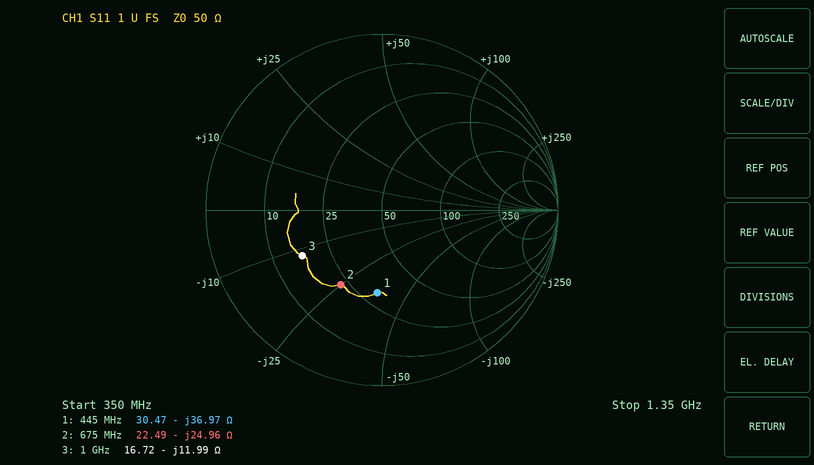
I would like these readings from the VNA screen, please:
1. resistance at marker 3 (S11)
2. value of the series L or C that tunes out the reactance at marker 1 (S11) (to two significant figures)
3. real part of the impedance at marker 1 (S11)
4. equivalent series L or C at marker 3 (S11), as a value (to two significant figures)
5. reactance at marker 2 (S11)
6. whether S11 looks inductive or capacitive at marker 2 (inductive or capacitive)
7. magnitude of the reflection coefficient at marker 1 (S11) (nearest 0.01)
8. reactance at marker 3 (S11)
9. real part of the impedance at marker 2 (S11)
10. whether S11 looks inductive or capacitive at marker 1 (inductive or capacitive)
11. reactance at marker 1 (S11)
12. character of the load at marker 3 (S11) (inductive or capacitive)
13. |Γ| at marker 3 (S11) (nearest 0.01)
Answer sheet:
16.72 Ω
13 nH
30.47 Ω
13 pF
-24.96 Ω
capacitive
0.47
-11.99 Ω
22.49 Ω
capacitive
-36.97 Ω
capacitive
0.52
